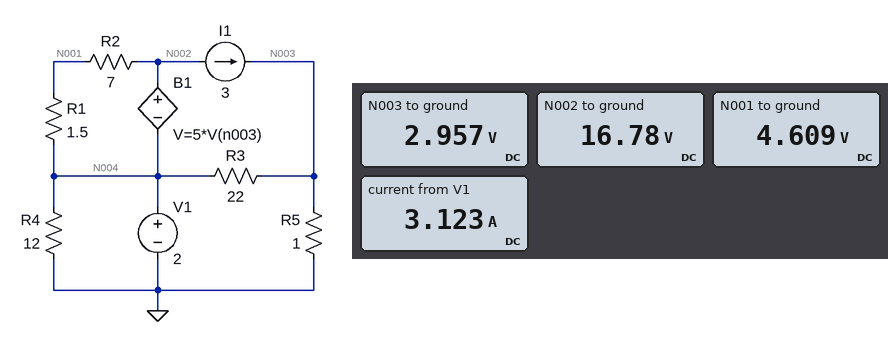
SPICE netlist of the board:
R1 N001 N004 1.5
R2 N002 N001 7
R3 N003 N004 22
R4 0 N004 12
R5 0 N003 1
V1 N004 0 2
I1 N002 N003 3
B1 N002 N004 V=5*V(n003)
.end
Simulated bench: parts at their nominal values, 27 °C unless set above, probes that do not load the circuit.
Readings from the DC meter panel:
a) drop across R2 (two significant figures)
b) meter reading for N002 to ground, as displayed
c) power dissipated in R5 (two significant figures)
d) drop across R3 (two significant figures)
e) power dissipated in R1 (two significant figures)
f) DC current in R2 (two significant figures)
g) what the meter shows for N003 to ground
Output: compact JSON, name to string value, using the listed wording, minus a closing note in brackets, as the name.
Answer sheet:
{"drop across R2": "12 V", "meter reading for N002 to ground, as displayed": "16.78 V", "power dissipated in R5": "8.7 W", "drop across R3": "960 mV", "power dissipated in R1": "4.5 W", "DC current in R2": "1.7 A", "what the meter shows for N003 to ground": "2.957 V"}
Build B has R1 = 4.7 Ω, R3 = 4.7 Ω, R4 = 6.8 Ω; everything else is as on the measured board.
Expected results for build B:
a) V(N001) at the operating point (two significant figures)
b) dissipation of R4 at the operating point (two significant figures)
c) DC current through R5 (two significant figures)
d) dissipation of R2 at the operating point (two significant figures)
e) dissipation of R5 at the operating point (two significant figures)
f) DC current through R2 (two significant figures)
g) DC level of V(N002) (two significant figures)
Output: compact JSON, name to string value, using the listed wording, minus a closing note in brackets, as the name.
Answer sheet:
{"V(N001) at the operating point": "7.7 V", "dissipation of R4 at the operating point": "590 mW", "DC current through R5": "2.8 A", "dissipation of R2 at the operating point": "10 W", "dissipation of R5 at the operating point": "8.0 W", "DC current through R2": "1.2 A", "DC level of V(N002)": "16 V"}
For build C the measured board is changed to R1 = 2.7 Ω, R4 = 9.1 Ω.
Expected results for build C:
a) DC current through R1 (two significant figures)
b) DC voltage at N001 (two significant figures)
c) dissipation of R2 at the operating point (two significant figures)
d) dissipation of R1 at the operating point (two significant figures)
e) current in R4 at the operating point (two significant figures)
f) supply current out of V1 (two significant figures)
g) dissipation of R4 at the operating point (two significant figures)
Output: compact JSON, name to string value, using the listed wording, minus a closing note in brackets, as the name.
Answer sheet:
{"DC current through R1": "1.5 A", "DC voltage at N001": "6.1 V", "dissipation of R2 at the operating point": "16 W", "dissipation of R1 at the operating point": "6.3 W", "current in R4 at the operating point": "220 mA", "supply current out of V1": "3.2 A", "dissipation of R4 at the operating point": "440 mW"}
